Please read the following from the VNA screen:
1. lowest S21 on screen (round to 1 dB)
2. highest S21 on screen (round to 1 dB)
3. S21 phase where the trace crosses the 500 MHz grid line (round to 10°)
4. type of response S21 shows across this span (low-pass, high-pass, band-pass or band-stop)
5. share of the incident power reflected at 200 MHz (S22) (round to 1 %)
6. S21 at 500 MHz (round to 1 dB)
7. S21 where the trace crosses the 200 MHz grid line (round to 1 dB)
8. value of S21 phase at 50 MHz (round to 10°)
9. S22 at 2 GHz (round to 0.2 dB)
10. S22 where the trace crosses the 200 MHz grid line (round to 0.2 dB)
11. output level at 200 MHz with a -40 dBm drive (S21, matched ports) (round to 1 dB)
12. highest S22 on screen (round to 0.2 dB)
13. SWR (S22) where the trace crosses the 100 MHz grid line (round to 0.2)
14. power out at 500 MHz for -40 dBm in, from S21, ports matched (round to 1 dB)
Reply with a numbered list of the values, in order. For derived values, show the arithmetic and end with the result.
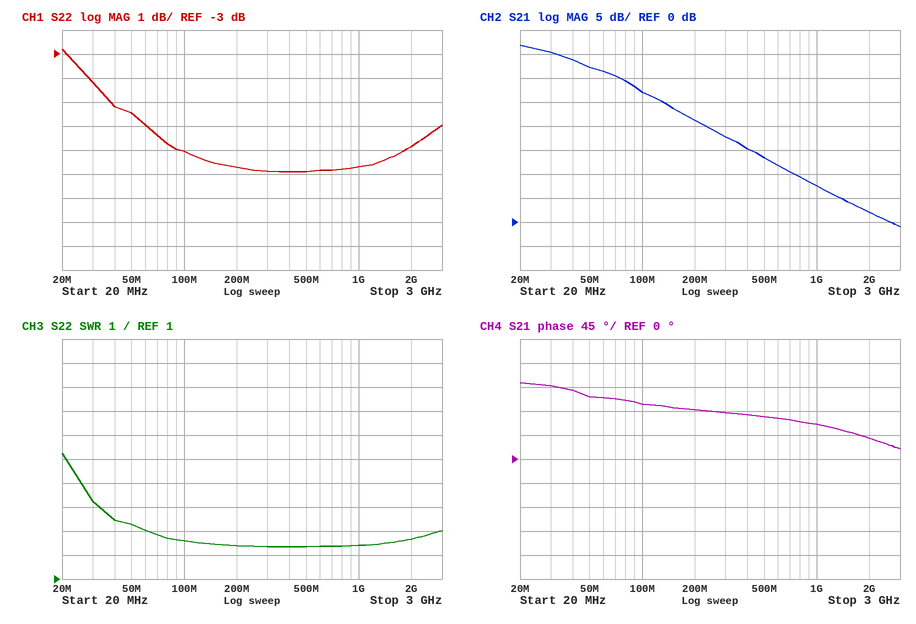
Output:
1. -1 dB
2. 37 dB
3. 80°
4. low-pass
5. 10^(-7.8/10) ≈ 17 %
6. 13 dB
7. 21 dB
8. 120°
9. -6.8 dB
10. -7.8 dB
11. -40 dBm + (21 dB) = -19 dBm
12. -2.8 dB
13. 2.6
14. -40 dBm + (13 dB) = -27 dBm
